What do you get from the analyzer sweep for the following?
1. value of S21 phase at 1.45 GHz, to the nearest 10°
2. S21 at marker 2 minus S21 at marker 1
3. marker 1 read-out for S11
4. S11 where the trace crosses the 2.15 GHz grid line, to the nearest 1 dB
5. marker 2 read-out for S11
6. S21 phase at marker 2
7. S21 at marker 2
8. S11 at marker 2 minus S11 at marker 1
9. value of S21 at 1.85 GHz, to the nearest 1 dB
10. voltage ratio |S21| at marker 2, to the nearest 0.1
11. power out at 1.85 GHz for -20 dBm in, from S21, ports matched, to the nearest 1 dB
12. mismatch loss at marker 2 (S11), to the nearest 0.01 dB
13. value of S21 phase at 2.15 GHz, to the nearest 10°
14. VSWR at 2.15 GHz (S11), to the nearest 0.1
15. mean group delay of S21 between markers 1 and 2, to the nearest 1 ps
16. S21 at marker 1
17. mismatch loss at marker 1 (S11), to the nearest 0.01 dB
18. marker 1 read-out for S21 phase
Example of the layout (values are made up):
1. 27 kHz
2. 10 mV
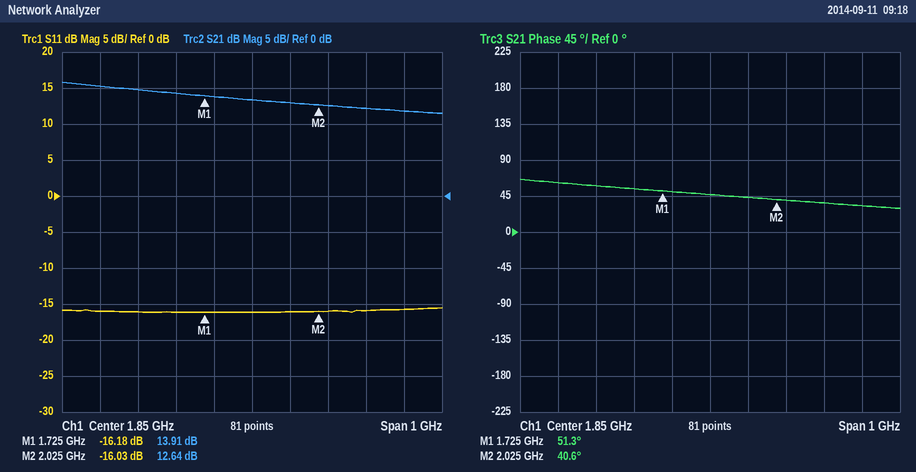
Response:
1. 60°
2. -1.27 dB
3. -16.18 dB
4. -16 dB
5. -16.03 dB
6. 40.6°
7. 12.64 dB
8. 0.15 dB
9. 13 dB
10. 4.3
11. -7 dBm
12. 0.11 dB
13. 40°
14. 1.4
15. 99 ps
16. 13.91 dB
17. 0.11 dB
18. 51.3°
